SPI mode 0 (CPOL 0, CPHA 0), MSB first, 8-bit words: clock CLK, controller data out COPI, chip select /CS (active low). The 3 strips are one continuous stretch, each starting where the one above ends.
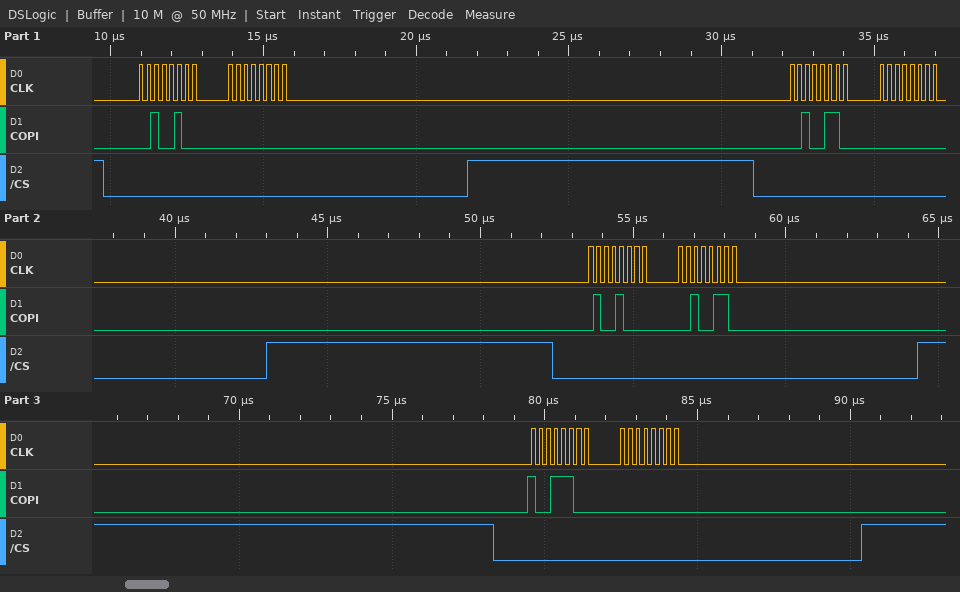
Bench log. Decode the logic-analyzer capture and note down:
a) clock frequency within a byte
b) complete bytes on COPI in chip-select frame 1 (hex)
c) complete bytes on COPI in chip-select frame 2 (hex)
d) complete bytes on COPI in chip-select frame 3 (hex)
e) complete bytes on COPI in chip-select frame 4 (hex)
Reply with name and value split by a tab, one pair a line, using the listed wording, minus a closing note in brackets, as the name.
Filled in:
clock frequency within a byte	4 MHz
complete bytes on COPI in chip-select frame 1	0x24 0x00
complete bytes on COPI in chip-select frame 2	0x26 0x00
complete bytes on COPI in chip-select frame 3	0x48 0x26
complete bytes on COPI in chip-select frame 4	0x9C 0x00
